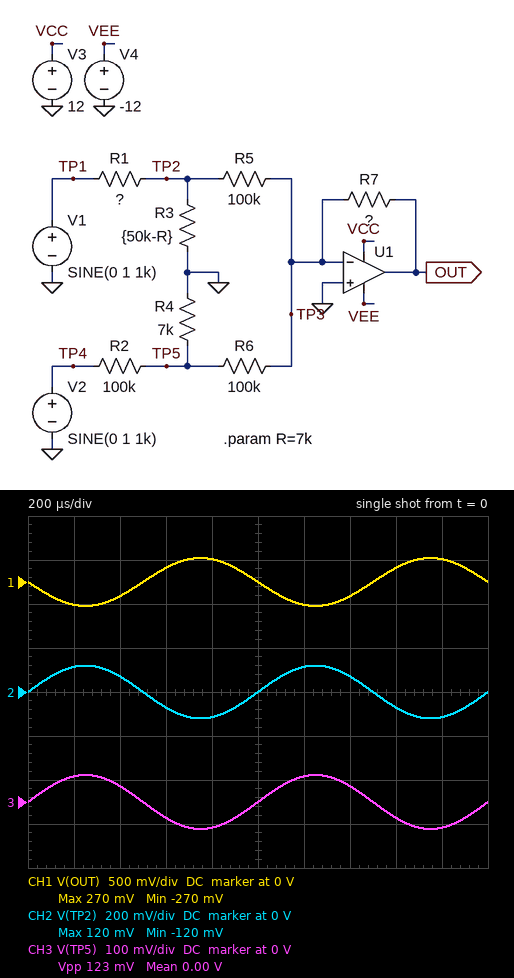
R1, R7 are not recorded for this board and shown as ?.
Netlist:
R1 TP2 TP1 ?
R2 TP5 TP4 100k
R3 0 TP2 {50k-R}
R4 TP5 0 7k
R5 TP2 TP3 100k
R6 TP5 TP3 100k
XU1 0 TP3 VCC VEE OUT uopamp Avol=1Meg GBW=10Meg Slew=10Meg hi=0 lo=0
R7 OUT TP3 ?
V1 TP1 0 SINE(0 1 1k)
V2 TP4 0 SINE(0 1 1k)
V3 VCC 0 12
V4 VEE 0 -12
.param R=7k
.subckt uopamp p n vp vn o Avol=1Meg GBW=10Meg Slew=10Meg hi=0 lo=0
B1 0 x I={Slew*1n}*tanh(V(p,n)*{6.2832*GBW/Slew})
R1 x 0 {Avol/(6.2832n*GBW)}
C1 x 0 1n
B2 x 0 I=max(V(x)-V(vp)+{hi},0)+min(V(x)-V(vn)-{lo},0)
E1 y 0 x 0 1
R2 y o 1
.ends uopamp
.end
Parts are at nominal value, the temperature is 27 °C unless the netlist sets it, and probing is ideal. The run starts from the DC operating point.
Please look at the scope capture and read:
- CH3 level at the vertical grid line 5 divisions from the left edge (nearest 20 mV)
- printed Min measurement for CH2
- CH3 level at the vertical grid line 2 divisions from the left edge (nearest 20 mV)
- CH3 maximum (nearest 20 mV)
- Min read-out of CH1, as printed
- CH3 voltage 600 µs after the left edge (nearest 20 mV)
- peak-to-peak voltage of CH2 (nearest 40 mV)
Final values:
0 V
-120 mV
40 mV
60 mV
-270 mV
-40 mV
240 mV
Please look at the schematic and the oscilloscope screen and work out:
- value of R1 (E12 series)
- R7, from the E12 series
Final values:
220 kΩ
150 kΩ
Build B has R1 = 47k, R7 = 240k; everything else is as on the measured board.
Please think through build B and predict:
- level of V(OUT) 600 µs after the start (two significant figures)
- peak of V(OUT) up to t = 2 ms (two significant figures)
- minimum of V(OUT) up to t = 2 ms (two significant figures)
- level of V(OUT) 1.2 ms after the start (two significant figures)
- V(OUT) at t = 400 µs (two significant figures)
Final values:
640 mV
1.1 V
-1.1 V
-1.0 V
-640 mV
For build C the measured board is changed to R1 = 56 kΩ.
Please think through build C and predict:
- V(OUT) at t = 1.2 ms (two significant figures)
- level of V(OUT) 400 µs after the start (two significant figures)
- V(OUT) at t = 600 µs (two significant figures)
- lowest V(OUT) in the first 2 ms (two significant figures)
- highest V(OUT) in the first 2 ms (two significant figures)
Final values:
-590 mV
-360 mV
360 mV
-620 mV
620 mV
